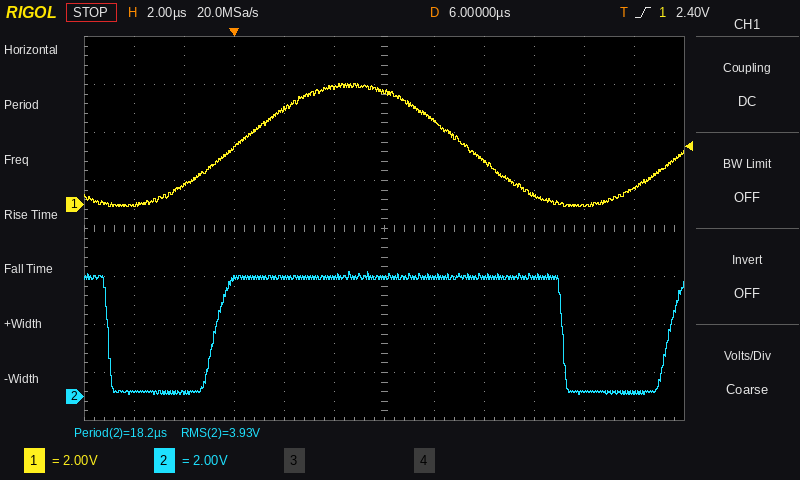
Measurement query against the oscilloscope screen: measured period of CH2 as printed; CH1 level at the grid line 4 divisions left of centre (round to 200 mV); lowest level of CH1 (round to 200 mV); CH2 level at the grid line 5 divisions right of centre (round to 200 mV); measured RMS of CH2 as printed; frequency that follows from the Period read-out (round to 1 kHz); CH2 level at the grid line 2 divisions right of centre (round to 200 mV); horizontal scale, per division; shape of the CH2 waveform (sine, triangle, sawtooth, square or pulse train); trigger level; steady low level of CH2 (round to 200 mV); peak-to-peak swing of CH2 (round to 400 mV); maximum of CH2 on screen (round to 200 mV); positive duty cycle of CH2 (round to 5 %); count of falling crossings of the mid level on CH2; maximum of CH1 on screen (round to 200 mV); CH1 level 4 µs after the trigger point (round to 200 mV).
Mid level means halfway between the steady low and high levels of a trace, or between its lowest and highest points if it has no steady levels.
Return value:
18.2 µs
800 mV
0.0 V
200 mV
3.93 V
55 kHz
5.0 V
2 µs
pulse train
2.40 V
200 mV
5.2 V
5.2 V
75 %
2
5.0 V
4.8 V
